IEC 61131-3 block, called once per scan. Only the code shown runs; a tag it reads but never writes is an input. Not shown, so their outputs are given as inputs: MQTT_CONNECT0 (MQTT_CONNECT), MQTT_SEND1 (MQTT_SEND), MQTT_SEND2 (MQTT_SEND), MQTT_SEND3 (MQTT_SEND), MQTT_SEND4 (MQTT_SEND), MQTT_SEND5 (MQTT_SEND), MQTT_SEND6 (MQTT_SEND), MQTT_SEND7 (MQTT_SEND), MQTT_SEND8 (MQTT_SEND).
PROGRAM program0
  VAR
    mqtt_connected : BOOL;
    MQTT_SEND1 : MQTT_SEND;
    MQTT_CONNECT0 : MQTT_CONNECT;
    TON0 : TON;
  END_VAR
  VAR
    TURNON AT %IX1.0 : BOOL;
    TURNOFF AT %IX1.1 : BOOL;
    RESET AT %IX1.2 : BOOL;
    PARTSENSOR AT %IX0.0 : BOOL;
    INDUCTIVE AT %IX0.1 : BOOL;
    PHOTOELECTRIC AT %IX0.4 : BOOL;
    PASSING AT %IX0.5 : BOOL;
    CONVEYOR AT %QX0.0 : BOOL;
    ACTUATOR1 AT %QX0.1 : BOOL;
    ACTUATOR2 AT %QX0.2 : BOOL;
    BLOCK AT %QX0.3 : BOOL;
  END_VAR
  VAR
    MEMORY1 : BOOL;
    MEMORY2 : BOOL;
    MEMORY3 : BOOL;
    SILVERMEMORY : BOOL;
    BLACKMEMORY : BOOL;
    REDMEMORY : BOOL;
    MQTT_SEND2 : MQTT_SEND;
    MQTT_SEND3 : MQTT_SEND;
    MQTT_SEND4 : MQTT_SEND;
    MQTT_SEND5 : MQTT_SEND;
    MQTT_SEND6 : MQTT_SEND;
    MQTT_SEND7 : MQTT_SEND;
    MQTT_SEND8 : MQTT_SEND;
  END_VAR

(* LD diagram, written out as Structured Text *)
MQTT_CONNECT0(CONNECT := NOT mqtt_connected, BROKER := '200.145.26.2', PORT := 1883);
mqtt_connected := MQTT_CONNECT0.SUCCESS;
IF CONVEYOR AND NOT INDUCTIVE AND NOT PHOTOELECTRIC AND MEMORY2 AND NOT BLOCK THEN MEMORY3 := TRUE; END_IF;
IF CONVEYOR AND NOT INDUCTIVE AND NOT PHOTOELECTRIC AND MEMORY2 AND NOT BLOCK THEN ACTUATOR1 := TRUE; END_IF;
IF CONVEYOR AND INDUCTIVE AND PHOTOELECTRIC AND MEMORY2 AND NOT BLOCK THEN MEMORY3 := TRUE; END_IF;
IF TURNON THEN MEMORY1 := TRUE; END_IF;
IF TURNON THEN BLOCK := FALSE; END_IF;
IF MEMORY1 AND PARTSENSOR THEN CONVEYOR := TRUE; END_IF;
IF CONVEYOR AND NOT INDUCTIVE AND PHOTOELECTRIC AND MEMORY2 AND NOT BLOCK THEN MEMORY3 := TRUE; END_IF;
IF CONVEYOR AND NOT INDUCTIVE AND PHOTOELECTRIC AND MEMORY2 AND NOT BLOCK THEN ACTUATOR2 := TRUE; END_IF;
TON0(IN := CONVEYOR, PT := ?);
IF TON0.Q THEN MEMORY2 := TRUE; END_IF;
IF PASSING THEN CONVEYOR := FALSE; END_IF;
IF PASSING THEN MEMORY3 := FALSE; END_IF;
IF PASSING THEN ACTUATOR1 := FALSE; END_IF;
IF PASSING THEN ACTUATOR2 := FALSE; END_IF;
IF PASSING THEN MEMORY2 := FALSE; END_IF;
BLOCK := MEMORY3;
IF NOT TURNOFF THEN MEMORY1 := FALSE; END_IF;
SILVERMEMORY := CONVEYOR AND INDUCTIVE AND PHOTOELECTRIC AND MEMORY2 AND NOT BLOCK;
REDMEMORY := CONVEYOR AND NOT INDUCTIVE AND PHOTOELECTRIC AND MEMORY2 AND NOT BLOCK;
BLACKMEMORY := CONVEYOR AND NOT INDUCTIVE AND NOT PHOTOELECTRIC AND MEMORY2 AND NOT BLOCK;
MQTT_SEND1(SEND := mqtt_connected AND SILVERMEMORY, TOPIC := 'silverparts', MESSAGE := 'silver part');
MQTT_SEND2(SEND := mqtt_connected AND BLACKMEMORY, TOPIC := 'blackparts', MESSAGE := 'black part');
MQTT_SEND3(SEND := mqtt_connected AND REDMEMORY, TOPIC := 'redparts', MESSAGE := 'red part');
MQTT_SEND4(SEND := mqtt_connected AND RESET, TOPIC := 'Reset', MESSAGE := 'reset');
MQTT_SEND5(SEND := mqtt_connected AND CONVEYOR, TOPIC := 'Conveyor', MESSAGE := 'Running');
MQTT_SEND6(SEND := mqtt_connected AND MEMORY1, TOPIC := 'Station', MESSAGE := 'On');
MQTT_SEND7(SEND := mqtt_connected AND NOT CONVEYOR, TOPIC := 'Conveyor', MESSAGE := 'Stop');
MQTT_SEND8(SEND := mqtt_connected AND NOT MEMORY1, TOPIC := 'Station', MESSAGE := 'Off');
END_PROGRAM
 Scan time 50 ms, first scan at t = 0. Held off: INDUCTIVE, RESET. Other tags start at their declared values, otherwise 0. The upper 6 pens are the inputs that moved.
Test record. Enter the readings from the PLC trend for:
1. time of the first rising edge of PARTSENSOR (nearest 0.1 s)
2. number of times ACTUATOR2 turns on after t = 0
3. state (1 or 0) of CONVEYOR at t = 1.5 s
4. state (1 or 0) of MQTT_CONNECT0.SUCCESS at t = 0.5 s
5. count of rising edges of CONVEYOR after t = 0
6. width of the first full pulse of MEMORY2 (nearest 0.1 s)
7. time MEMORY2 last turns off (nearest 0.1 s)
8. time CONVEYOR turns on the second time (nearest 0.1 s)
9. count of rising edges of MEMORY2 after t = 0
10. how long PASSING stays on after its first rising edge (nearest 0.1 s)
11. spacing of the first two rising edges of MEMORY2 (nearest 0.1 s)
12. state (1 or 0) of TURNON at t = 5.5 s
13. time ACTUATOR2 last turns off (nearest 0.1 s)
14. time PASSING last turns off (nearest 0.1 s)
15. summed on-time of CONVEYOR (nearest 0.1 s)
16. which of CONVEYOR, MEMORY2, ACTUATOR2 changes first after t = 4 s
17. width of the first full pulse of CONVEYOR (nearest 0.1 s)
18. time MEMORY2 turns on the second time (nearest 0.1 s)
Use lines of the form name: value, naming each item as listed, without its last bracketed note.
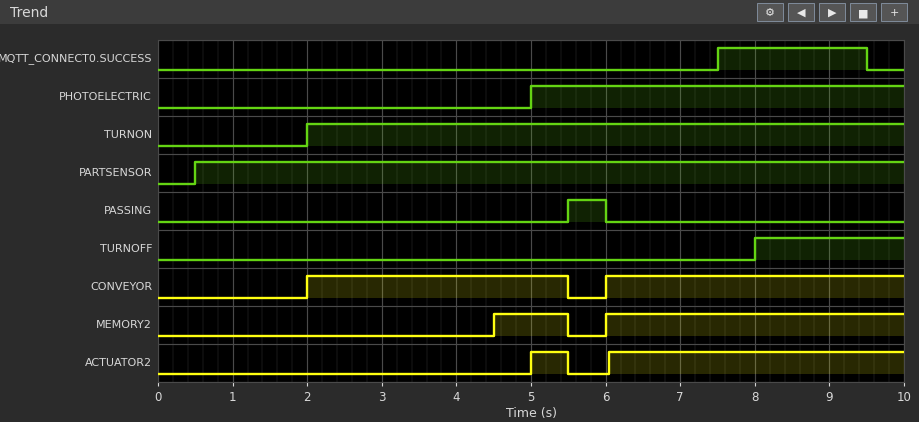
time of the first rising edge of PARTSENSOR: 0.5 s
number of times ACTUATOR2 turns on after t = 0: 2
state (1 or 0) of CONVEYOR at t = 1.5 s: 0
state (1 or 0) of MQTT_CONNECT0.SUCCESS at t = 0.5 s: 0
count of rising edges of CONVEYOR after t = 0: 2
width of the first full pulse of MEMORY2: 1.0 s
time MEMORY2 last turns off: 5.5 s
time CONVEYOR turns on the second time: 6.0 s
count of rising edges of MEMORY2 after t = 0: 2
how long PASSING stays on after its first rising edge: 0.5 s
spacing of the first two rising edges of MEMORY2: 1.5 s
state (1 or 0) of TURNON at t = 5.5 s: 1
time ACTUATOR2 last turns off: 5.5 s
time PASSING last turns off: 6.0 s
summed on-time of CONVEYOR: 7.5 s
which of CONVEYOR, MEMORY2, ACTUATOR2 changes first after t = 4 s: MEMORY2
width of the first full pulse of CONVEYOR: 3.5 s
time MEMORY2 turns on the second time: 6.0 s
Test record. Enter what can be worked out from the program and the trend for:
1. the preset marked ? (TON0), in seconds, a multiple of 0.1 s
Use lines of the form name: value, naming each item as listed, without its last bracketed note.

the preset marked ? (TON0), in seconds, a multiple of 0.1 s: 2.5 s
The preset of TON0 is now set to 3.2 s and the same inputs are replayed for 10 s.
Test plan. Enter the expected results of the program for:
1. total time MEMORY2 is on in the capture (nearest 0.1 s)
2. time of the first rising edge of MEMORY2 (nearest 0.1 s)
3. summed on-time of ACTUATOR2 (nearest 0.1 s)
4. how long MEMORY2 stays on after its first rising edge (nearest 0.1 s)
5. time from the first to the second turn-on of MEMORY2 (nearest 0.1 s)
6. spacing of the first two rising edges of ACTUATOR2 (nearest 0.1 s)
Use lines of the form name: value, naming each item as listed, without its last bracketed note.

total time MEMORY2 is on in the capture: 4.3 s
time of the first rising edge of MEMORY2: 5.2 s
summed on-time of ACTUATOR2: 4.2 s
how long MEMORY2 stays on after its first rising edge: 0.3 s
time from the first to the second turn-on of MEMORY2: 0.8 s
spacing of the first two rising edges of ACTUATOR2: 0.8 s
